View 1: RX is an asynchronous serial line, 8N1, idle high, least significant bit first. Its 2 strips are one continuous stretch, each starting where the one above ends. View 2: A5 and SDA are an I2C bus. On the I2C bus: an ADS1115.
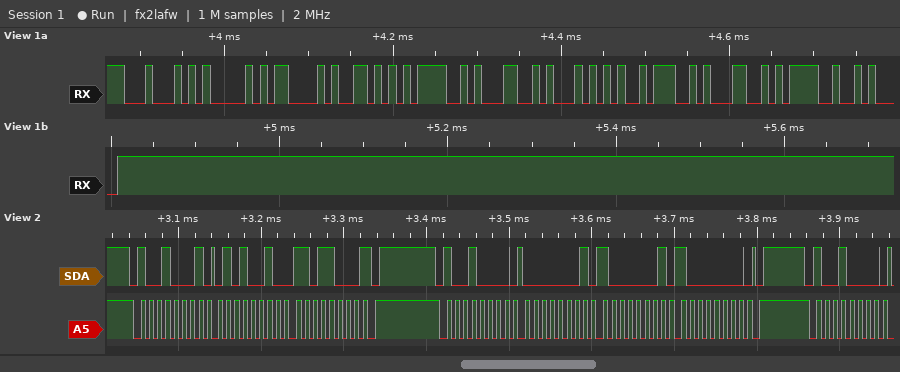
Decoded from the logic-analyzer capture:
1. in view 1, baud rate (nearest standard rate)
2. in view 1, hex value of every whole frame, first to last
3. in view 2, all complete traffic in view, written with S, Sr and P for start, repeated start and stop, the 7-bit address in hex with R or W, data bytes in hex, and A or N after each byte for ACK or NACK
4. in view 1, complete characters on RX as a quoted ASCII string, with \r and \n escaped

115200 baud
44 41 43 56 4F 4C 54 3A 31 3D 0A
S 48R A 52 A D8 N P S 48W A 01 A 81 A 80 A P S 48W A
"DACVOLT:1=\n"
